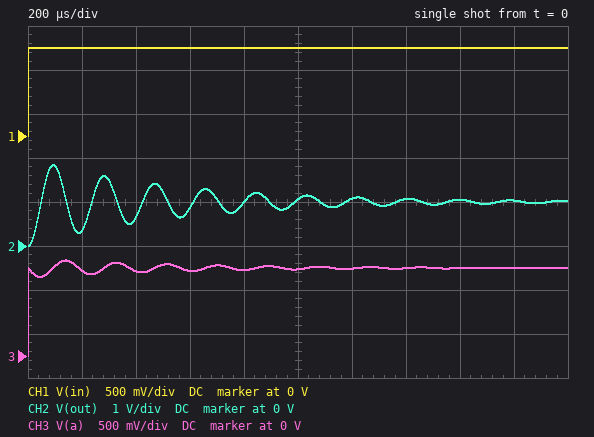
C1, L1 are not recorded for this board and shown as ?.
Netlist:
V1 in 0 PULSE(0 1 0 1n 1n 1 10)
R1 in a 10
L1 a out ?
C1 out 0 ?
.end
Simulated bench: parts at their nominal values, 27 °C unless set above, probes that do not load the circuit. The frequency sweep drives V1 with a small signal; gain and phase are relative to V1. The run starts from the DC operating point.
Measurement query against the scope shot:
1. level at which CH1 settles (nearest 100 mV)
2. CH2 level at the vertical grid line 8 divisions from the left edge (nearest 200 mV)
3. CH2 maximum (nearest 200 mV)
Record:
1.0 V
1.0 V
1.8 V
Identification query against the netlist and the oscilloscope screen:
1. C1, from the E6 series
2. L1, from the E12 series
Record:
330 nF
2.7 mH
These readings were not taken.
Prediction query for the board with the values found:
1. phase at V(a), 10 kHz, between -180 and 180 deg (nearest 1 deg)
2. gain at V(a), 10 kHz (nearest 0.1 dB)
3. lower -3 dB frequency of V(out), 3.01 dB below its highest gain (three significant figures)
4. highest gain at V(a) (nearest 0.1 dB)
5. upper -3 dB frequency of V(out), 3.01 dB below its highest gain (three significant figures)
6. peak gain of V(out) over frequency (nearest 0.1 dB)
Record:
5 deg
0 dB
5.01 kHz
0 dB
5.60 kHz
19.1 dB
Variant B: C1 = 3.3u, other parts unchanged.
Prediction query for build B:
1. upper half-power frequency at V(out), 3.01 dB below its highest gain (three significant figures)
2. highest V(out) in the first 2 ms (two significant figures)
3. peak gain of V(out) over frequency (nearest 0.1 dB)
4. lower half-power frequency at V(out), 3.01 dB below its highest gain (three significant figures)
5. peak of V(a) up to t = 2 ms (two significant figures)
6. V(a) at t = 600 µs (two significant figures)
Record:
1.91 kHz
1.6 V
9.3 dB
1.30 kHz
1.2 V
1.0 V
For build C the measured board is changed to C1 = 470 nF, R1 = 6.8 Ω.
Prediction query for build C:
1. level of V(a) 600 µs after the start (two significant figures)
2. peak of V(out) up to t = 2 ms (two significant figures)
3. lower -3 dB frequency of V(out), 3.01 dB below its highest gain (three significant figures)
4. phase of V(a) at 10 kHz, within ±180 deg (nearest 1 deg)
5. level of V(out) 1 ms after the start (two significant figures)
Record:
1.0 V
1.9 V
4.25 kHz
3 deg
1.3 V
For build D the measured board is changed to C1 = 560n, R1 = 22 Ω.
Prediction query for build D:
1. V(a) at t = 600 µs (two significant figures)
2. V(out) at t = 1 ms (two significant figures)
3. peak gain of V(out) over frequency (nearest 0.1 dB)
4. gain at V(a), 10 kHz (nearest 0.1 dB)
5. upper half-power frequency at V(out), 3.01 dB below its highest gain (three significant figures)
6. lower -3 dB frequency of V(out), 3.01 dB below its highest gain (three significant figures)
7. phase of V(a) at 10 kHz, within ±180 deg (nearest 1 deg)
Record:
990 mV
980 mV
10.1 dB
-0.1 dB
4.60 kHz
3.27 kHz
9 deg
